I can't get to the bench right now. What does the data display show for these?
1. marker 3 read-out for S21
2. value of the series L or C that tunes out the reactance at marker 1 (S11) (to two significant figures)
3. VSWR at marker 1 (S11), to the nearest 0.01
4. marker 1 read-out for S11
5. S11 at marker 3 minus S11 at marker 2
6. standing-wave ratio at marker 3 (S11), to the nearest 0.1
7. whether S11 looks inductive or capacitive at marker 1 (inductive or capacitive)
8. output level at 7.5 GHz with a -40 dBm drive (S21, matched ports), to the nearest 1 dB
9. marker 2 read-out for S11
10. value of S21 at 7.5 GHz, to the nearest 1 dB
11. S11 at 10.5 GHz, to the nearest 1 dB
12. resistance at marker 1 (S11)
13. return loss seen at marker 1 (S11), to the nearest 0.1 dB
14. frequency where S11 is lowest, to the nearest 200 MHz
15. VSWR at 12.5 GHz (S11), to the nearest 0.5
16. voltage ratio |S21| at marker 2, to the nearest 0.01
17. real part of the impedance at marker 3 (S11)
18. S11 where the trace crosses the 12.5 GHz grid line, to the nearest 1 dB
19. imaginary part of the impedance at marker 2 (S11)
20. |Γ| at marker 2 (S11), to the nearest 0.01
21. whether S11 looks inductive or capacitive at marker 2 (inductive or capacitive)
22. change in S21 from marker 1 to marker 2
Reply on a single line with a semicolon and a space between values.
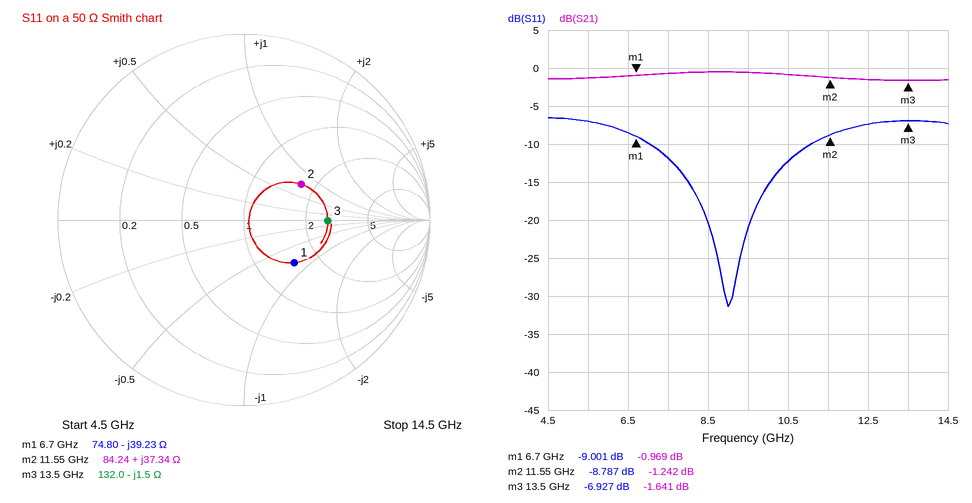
-1.641 dB; 930 pH; 2.10; -9.001 dB; 1.860 dB; 2.6; capacitive; -41 dBm; -8.787 dB; -1 dB; -12 dB; 74.80 Ω; 9.0 dB; 9.0 GHz; 2.5; 0.87; 132.0 Ω; -7 dB; +37.34 Ω; 0.36; inductive; -0.273 dB
